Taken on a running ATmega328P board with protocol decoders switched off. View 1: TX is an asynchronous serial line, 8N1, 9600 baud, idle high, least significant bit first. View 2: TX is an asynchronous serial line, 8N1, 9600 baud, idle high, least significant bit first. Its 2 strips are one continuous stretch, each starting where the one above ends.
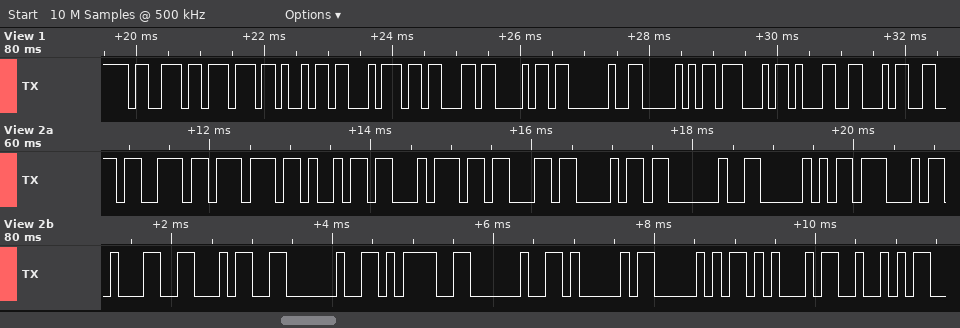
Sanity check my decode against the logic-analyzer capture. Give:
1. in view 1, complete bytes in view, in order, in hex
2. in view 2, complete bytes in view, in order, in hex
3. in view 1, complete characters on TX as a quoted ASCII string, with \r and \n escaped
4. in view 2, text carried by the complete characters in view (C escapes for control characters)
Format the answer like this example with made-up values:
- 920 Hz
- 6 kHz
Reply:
- 73 77 69 74 63 68 20 50 47 31 34
- 0x73 0x77 0x69 0x74 0x63 0x68 0x20 0x50 0x47 0x31 0x34 0x20 0x3D 0x20 0x41 0x50 0x45 0x52
- "switch PG14"
- "switch PG14 = APER"
